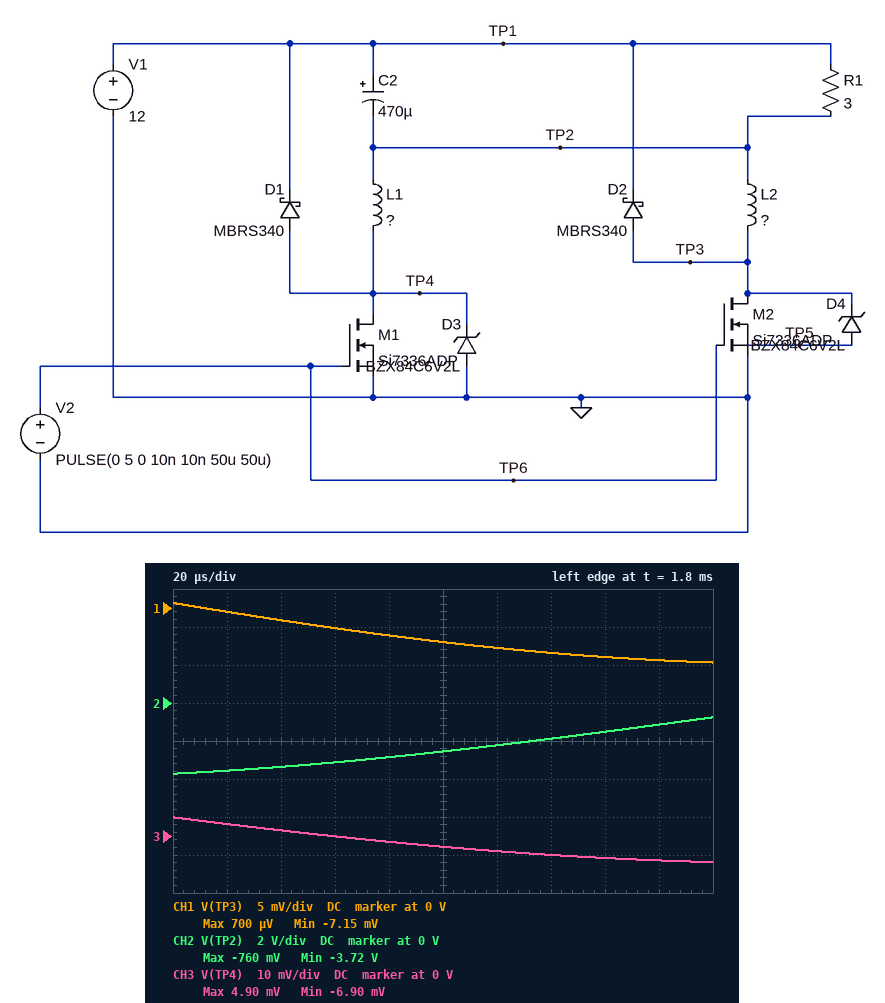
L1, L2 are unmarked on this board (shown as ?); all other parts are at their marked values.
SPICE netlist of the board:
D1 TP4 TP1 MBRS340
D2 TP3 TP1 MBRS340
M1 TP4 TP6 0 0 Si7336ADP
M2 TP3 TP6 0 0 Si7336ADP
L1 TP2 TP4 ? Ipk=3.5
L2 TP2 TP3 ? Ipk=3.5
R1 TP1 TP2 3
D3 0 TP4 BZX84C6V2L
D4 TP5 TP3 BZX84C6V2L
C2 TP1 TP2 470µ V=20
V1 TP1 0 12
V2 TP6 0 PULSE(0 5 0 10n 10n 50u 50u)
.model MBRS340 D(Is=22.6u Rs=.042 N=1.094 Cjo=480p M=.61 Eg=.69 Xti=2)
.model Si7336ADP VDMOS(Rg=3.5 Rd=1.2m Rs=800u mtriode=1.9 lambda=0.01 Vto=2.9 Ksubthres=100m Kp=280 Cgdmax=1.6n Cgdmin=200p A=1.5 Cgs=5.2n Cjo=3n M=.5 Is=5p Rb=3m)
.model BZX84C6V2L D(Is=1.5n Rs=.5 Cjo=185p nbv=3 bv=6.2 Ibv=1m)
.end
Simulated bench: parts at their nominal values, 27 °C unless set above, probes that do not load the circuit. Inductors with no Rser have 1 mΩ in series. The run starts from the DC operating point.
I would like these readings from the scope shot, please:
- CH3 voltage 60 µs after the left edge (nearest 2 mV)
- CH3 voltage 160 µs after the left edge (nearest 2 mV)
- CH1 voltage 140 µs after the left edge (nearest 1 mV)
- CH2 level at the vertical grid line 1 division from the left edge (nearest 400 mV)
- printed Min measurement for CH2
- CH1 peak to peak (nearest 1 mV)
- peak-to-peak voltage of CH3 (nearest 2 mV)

0 V
-6 mV
-6 mV
-3.6 V
-3.72 V
8 mV
12 mV
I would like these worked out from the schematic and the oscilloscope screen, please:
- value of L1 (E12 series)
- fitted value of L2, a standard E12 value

120 µH
180 µH
